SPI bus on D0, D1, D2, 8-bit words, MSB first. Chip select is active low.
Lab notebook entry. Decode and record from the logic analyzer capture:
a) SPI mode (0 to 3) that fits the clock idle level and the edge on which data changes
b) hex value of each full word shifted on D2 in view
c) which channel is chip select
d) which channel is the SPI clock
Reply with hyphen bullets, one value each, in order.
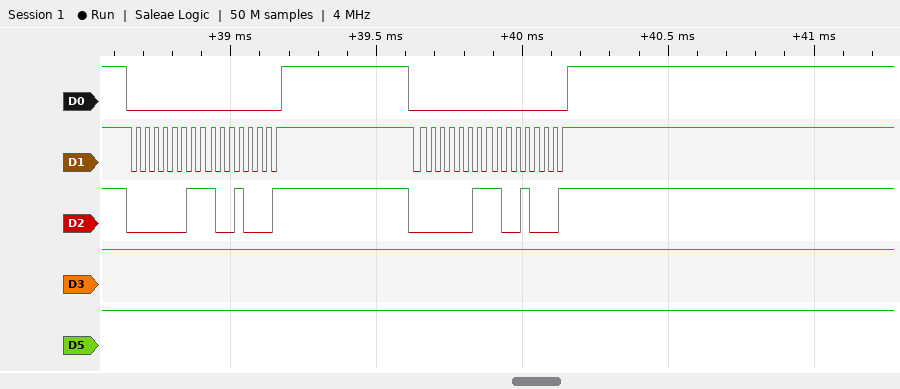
- 3
- 03, 91, 03, 91
- D0
- D1
